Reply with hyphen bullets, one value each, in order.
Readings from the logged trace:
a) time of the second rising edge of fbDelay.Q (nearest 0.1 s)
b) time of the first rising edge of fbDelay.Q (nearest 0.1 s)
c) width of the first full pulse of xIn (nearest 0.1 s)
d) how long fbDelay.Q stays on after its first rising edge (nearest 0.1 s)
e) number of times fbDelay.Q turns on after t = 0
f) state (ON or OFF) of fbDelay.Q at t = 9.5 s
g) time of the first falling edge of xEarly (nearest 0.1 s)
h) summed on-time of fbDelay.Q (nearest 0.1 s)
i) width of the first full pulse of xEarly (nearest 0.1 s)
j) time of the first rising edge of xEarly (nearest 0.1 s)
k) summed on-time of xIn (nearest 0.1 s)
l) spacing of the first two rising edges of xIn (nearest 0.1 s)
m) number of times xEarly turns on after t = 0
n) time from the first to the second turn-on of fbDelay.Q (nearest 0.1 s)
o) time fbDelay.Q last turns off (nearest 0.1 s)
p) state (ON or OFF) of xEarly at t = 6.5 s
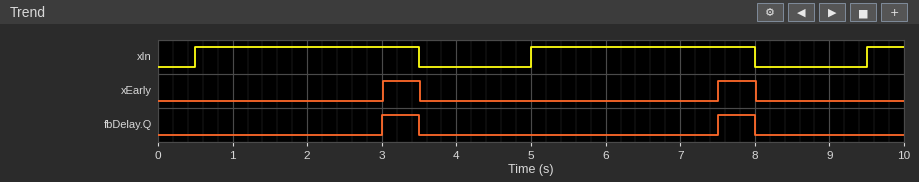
- 7.5 s
- 3.0 s
- 3.0 s
- 0.5 s
- 2
- OFF
- 3.5 s
- 1.0 s
- 0.5 s
- 3.0 s
- 6.5 s
- 4.5 s
- 2
- 4.5 s
- 8.0 s
- OFF
